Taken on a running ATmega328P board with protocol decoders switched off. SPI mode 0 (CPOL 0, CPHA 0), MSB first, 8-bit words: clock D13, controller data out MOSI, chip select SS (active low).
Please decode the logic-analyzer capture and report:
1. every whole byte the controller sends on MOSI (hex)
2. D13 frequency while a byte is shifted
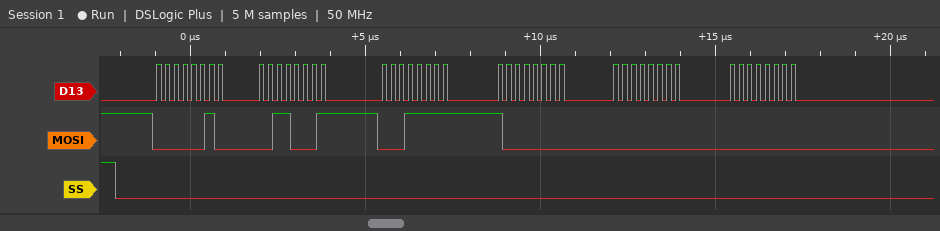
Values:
0x02 0x31 0x1F 0x80 0x00 0x00
4 MHz
